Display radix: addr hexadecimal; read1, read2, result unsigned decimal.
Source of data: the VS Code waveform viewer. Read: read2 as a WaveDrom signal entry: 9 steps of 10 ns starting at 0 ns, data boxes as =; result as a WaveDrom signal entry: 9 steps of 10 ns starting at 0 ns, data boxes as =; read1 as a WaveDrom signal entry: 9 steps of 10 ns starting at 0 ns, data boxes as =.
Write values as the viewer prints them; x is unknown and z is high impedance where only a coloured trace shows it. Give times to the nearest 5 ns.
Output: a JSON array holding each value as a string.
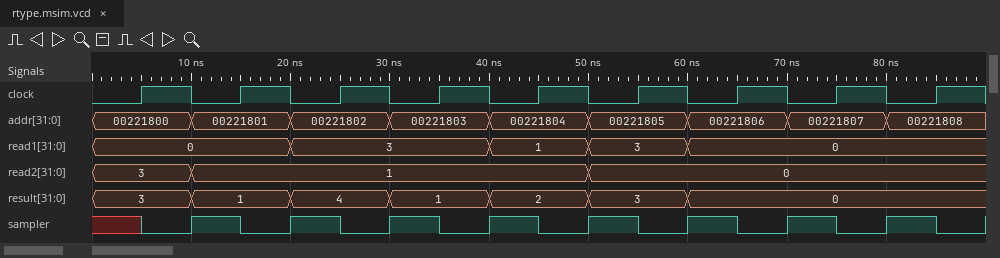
["{name: 'read2', wave: '==...=...', data: '3 1 0'}", "{name: 'result', wave: '=======..', data: '3 1 4 1 2 3 0'}", "{name: 'read1', wave: '=.=.===..', data: '0 3 1 3 0'}"]
